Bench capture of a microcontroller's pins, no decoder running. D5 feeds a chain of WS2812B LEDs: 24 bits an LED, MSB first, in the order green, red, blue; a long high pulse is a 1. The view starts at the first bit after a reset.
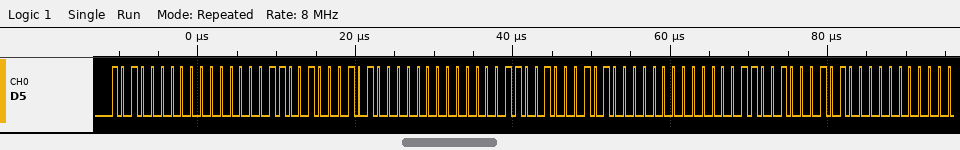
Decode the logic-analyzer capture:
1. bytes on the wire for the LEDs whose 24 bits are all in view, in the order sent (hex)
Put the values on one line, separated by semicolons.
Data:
A0 00 C8 A0 00 C8 A0 00 C8
